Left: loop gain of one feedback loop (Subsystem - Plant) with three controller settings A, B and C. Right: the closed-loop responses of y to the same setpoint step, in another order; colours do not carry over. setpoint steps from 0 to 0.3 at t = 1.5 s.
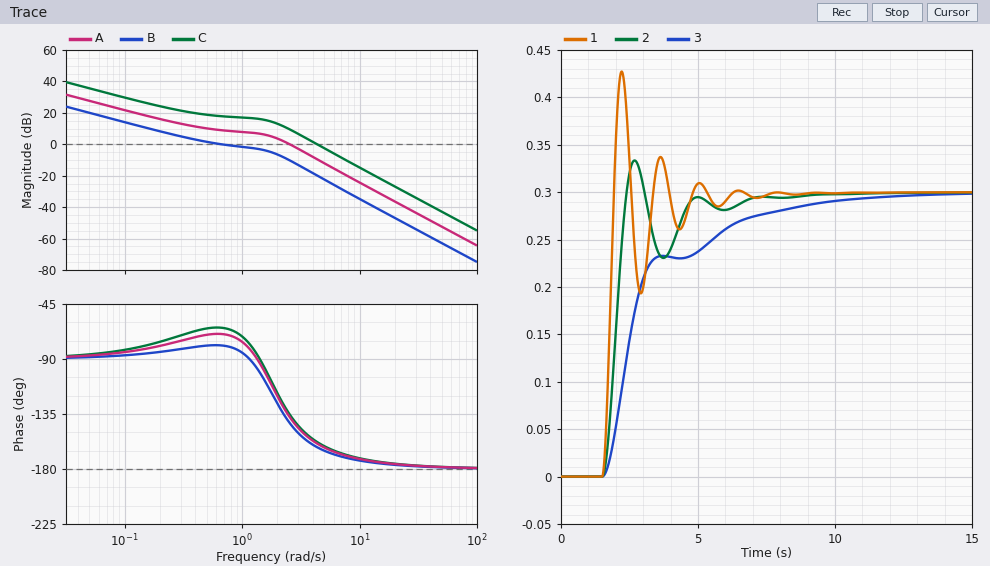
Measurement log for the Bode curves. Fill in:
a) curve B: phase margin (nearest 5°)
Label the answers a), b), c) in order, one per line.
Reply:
a) 100°
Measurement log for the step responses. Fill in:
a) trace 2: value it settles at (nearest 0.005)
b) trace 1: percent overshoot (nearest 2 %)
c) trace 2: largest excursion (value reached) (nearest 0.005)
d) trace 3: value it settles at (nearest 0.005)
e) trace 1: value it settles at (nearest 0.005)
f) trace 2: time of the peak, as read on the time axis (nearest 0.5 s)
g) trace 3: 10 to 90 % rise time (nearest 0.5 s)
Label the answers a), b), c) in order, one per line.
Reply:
a) 0.300
b) 42 %
c) 0.335
d) 0.300
e) 0.300
f) 2.5 s
g) 4.5 s
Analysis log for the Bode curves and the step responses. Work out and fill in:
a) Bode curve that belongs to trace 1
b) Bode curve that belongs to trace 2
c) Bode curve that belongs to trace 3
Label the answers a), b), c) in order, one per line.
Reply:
a) C
b) A
c) B
